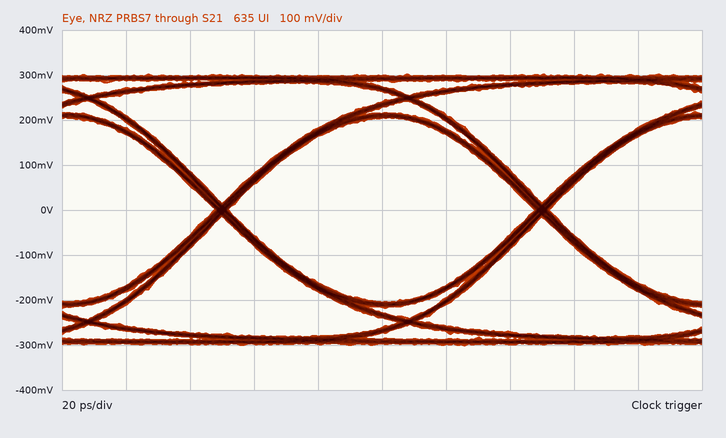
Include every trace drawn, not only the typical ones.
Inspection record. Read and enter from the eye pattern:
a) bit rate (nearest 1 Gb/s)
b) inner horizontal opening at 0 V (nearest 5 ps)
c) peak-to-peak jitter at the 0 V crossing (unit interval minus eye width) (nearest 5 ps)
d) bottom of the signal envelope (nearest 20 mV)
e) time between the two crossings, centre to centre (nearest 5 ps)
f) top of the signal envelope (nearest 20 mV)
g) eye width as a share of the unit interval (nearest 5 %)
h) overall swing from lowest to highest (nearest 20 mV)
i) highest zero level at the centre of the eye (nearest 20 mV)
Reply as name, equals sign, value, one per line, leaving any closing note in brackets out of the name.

bit rate = 10 Gb/s
inner horizontal opening at 0 V = 95 ps
peak-to-peak jitter at the 0 V crossing (unit interval minus eye width) = 5 ps
bottom of the signal envelope = -300 mV
time between the two crossings, centre to centre = 100 ps
top of the signal envelope = 300 mV
eye width as a share of the unit interval = 95 %
overall swing from lowest to highest = 600 mV
highest zero level at the centre of the eye = -200 mV
